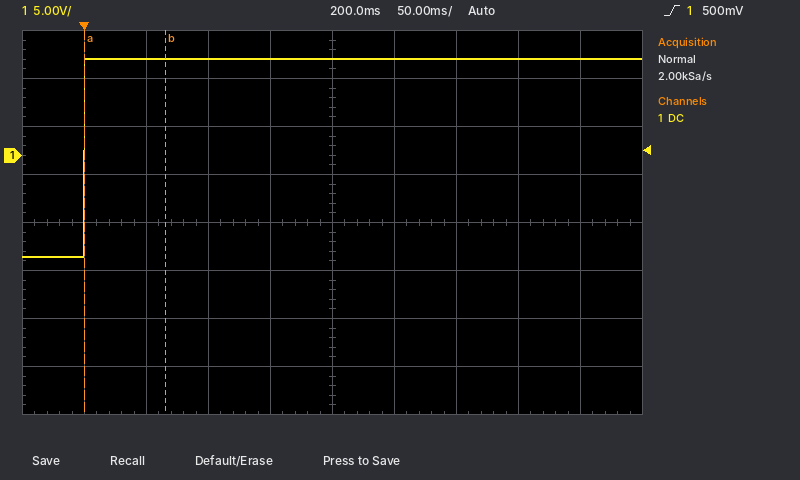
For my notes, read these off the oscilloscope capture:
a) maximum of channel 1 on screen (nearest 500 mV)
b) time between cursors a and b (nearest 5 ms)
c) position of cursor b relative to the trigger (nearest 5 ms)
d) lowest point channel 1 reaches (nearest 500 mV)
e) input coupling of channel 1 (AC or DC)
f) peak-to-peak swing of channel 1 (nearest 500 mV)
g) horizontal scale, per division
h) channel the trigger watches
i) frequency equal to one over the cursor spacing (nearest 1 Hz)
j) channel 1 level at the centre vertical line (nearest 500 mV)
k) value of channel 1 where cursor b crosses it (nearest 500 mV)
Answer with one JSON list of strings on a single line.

["10.0 V", "65 ms", "+65 ms", "-10.5 V", "DC", "20.5 V", "50 ms", "channel 1", "15 Hz", "10.0 V", "10.0 V"]
